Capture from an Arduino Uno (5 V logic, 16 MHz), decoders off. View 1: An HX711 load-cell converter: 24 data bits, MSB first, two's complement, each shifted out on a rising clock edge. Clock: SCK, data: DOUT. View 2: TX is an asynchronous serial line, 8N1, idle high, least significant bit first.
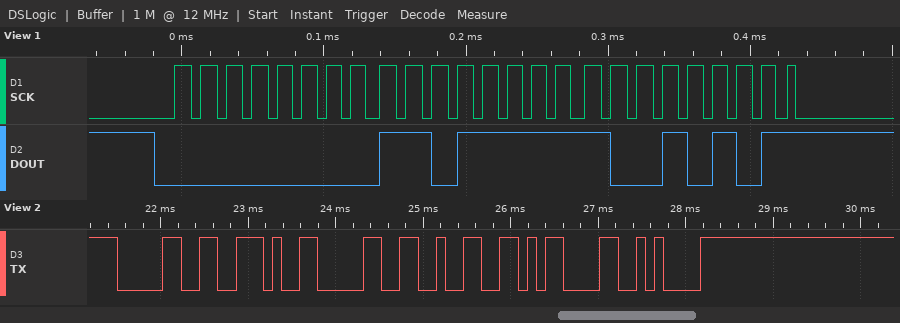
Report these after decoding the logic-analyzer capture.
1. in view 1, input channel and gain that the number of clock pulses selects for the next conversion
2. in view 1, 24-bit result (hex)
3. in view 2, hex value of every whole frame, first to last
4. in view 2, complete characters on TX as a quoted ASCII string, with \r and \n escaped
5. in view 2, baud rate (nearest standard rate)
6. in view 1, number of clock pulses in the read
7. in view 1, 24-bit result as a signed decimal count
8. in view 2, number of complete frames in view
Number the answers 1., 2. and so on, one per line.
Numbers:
1. channel A, gain 128
2. 0x00DF95
3. 0x30 0x2E 0x30 0x32 0x0D 0x0A
4. "0.02\r\n"
5. 9600 baud
6. 25
7. 57237
8. 6
